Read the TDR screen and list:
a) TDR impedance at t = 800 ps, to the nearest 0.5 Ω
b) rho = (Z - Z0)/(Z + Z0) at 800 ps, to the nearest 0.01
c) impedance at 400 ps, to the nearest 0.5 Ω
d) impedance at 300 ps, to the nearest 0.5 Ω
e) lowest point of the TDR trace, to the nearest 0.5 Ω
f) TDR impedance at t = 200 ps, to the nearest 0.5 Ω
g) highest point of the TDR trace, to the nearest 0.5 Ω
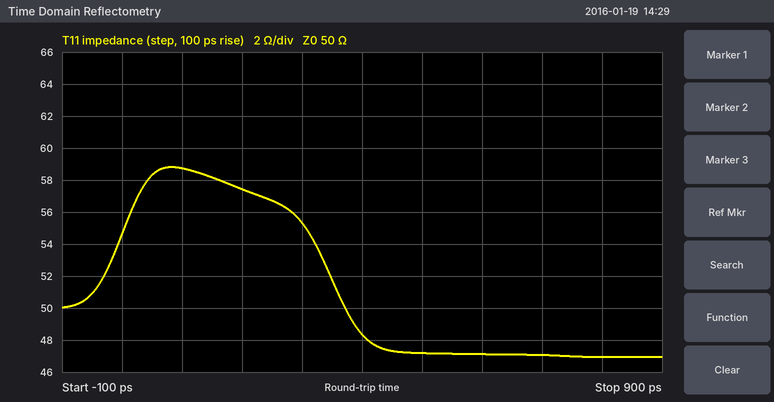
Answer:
47.0 Ω
-0.03
48.5 Ω
55.5 Ω
47.0 Ω
57.5 Ω
59.0 Ω
